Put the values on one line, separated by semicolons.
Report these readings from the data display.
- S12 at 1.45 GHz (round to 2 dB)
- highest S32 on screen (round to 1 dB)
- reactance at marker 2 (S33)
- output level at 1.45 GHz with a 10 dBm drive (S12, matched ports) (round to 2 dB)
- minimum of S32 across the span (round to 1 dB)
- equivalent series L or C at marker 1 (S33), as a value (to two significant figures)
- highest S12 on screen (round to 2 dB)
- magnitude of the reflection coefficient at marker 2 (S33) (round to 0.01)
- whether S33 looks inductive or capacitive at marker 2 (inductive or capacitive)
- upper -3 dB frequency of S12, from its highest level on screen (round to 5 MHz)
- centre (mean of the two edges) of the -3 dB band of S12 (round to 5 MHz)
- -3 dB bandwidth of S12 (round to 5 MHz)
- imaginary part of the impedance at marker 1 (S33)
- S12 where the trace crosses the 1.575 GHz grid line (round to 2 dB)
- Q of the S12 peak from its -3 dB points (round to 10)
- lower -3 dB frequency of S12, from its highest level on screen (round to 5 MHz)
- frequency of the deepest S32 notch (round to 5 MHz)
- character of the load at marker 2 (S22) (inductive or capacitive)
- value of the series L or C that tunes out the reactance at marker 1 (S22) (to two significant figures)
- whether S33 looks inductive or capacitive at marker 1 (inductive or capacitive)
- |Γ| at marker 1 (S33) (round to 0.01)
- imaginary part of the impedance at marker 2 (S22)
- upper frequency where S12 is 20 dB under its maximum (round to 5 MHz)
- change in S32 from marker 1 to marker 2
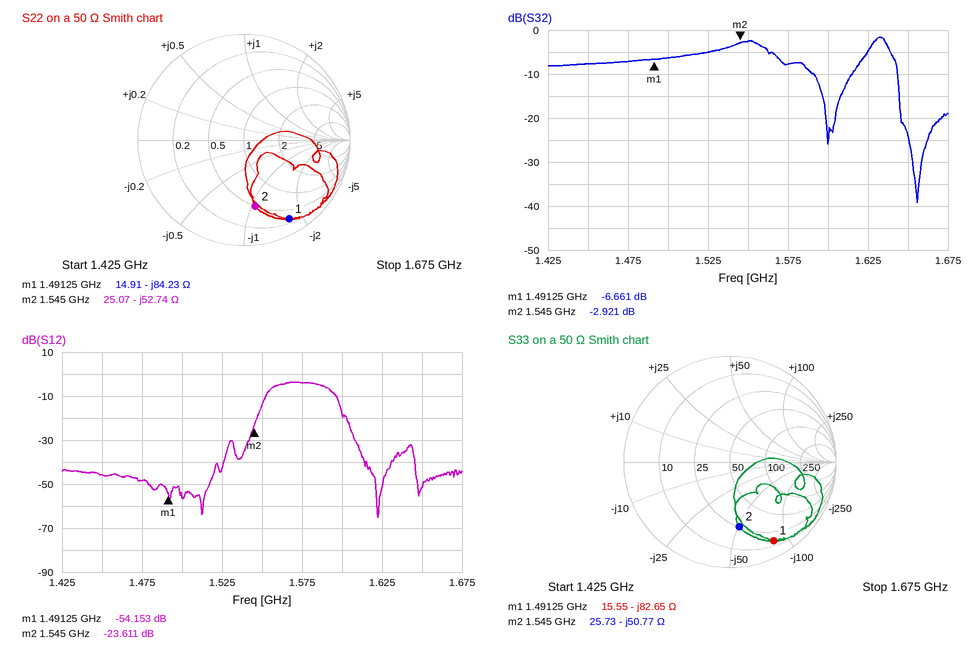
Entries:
-46 dB; -2 dB; -50.77 Ω; -36 dBm; -39 dB; 1.3 pF; -4 dB; 0.62; capacitive; 1.590 GHz; 1.575 GHz; 35 MHz; -82.65 Ω; -4 dB; 40; 1.555 GHz; 1.655 GHz; capacitive; 9.0 nH; capacitive; 0.85; -52.74 Ω; 1.605 GHz; 3.740 dB
